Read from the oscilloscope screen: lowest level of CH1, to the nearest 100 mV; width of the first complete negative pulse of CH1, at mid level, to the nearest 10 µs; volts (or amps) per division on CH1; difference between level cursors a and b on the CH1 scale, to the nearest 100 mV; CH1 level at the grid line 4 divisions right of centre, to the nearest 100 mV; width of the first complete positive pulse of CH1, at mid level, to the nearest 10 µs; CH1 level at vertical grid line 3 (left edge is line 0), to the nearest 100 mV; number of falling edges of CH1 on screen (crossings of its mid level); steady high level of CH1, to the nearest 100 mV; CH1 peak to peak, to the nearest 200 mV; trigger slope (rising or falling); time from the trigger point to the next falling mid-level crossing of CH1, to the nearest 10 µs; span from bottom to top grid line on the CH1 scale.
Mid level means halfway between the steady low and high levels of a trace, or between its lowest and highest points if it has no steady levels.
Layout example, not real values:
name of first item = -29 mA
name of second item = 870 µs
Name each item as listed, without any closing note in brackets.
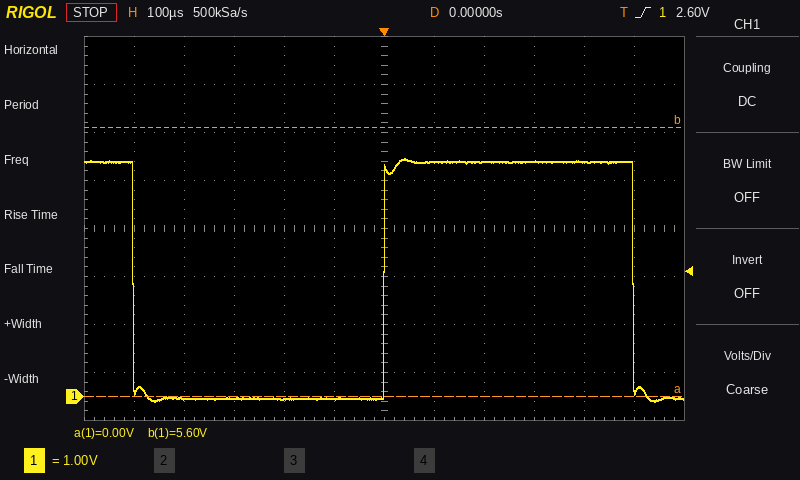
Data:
lowest level of CH1, to the nearest 100 mV = -100 mV
width of the first complete negative pulse of CH1, at mid level, to the nearest 10 µs = 500 µs
volts (or amps) per division on CH1 = 1 V
difference between level cursors a and b on the CH1 scale, to the nearest 100 mV = 5.6 V
CH1 level at the grid line 4 divisions right of centre, to the nearest 100 mV = 4.9 V
width of the first complete positive pulse of CH1, at mid level, to the nearest 10 µs = 500 µs
CH1 level at vertical grid line 3 (left edge is line 0), to the nearest 100 mV = 0.0 V
number of falling edges of CH1 on screen = 2
steady high level of CH1, to the nearest 100 mV = 4.9 V
CH1 peak to peak, to the nearest 200 mV = 5.0 V
trigger slope = rising
time from the trigger point to the next falling mid-level crossing of CH1, to the nearest 10 µs = 500 µs
span from bottom to top grid line on the CH1 scale = 8 V
